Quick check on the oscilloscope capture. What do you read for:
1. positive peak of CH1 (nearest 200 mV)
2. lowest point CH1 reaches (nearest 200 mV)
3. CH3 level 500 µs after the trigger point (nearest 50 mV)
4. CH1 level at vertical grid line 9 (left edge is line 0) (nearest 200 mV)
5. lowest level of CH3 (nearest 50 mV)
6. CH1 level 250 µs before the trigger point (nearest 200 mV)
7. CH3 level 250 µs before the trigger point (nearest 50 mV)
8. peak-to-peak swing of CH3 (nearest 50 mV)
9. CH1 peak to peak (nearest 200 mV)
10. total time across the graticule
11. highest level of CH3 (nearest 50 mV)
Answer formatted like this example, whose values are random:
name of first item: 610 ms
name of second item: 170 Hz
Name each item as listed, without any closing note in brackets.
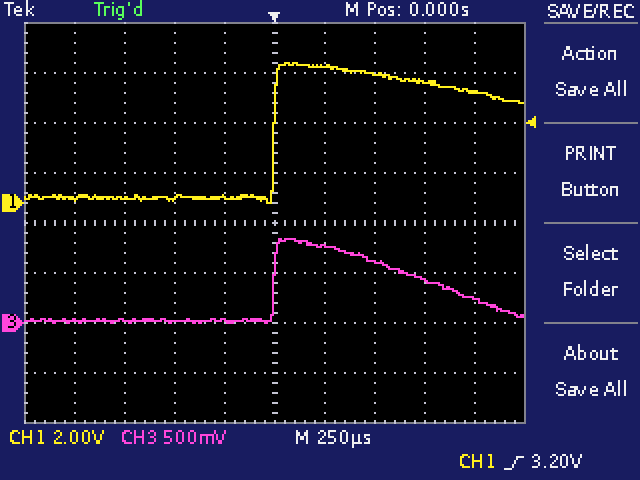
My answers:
positive peak of CH1: 5.6 V
lowest point CH1 reaches: 0.0 V
CH3 level 500 µs after the trigger point: 600 mV
CH1 level at vertical grid line 9 (left edge is line 0): 4.4 V
lowest level of CH3: 0 mV
CH1 level 250 µs before the trigger point: 200 mV
CH3 level 250 µs before the trigger point: 0 mV
peak-to-peak swing of CH3: 850 mV
CH1 peak to peak: 5.6 V
total time across the graticule: 2.5 ms
highest level of CH3: 850 mV
